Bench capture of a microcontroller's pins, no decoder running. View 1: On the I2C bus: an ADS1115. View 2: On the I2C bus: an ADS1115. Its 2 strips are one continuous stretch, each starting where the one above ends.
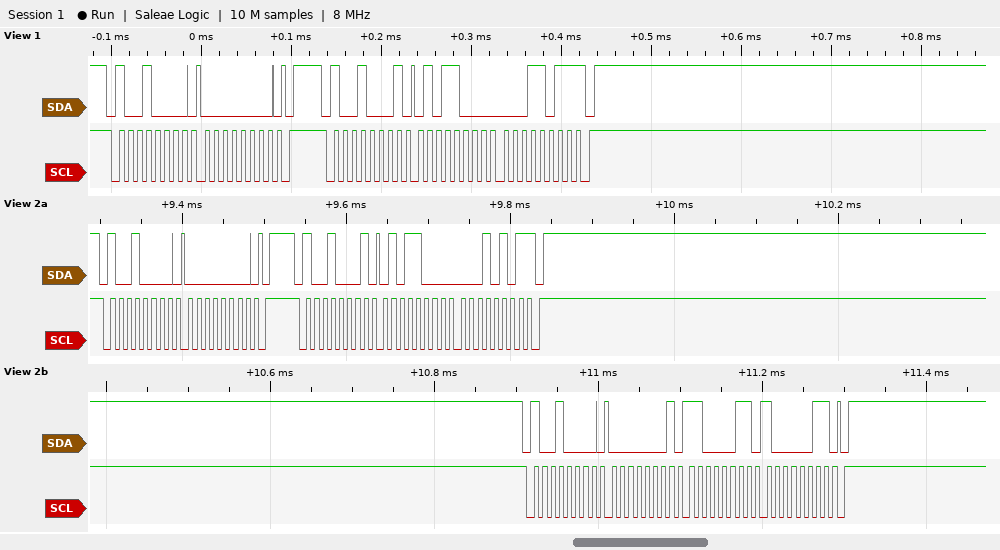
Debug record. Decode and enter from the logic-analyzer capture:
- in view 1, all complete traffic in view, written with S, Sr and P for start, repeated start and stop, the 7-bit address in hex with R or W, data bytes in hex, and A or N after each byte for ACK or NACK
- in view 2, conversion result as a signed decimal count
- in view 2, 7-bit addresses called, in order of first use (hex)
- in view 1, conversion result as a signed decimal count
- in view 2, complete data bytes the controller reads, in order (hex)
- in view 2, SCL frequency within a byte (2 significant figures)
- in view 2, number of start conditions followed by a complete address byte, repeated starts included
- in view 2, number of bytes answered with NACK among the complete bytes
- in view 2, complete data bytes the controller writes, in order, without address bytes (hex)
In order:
S 48W A 00 A P S 48R A 58 A 1B N P
22549
0x48
22555
58 15
100 kHz
3
1
00 01 C3 83
